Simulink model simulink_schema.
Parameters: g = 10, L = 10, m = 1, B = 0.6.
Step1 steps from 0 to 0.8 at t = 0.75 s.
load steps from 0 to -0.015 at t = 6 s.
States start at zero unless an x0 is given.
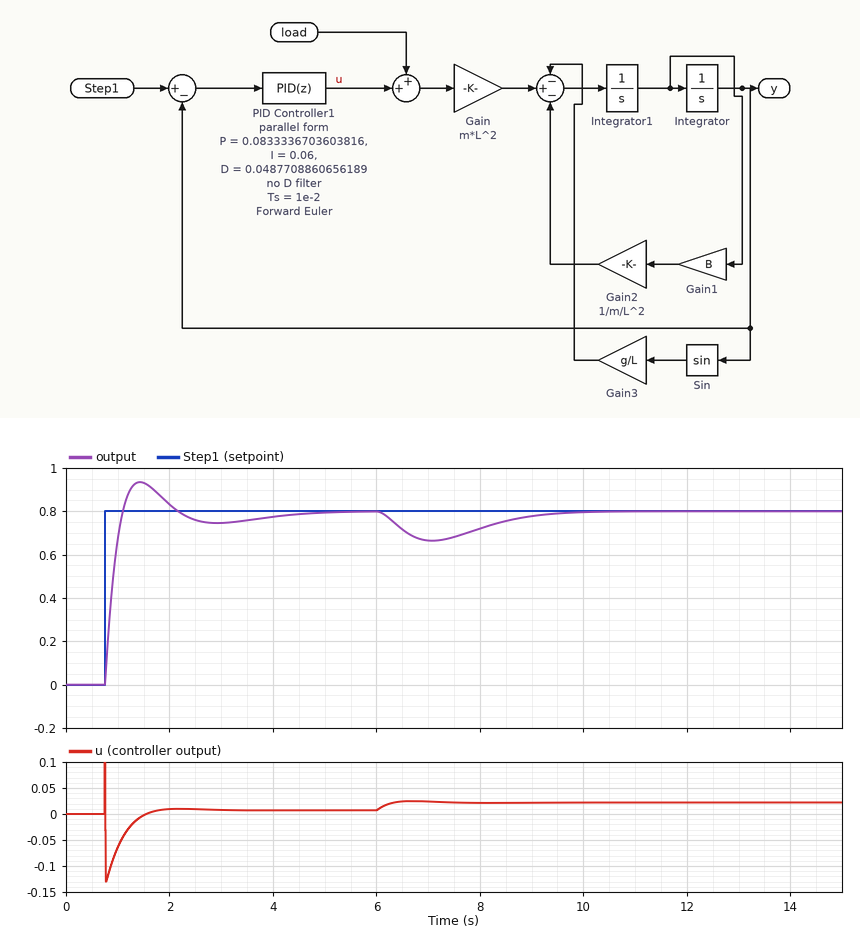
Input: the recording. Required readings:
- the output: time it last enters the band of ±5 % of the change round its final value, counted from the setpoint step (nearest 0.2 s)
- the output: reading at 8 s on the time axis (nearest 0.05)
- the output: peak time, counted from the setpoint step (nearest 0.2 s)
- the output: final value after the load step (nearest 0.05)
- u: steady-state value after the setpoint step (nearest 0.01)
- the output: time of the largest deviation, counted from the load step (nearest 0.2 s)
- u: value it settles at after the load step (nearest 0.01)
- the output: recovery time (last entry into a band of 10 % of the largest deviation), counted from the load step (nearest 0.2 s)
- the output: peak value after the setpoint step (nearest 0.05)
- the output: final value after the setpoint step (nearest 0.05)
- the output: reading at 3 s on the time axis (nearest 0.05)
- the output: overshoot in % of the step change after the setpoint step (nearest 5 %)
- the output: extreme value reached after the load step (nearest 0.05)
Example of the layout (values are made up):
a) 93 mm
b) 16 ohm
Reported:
a) 2.8 s
b) 0.70
c) 0.6 s
d) 0.80
e) 0.01
f) 1.0 s
g) 0.02
h) 3.4 s
i) 0.95
j) 0.80
k) 0.75
l) 15 %
m) 0.65
